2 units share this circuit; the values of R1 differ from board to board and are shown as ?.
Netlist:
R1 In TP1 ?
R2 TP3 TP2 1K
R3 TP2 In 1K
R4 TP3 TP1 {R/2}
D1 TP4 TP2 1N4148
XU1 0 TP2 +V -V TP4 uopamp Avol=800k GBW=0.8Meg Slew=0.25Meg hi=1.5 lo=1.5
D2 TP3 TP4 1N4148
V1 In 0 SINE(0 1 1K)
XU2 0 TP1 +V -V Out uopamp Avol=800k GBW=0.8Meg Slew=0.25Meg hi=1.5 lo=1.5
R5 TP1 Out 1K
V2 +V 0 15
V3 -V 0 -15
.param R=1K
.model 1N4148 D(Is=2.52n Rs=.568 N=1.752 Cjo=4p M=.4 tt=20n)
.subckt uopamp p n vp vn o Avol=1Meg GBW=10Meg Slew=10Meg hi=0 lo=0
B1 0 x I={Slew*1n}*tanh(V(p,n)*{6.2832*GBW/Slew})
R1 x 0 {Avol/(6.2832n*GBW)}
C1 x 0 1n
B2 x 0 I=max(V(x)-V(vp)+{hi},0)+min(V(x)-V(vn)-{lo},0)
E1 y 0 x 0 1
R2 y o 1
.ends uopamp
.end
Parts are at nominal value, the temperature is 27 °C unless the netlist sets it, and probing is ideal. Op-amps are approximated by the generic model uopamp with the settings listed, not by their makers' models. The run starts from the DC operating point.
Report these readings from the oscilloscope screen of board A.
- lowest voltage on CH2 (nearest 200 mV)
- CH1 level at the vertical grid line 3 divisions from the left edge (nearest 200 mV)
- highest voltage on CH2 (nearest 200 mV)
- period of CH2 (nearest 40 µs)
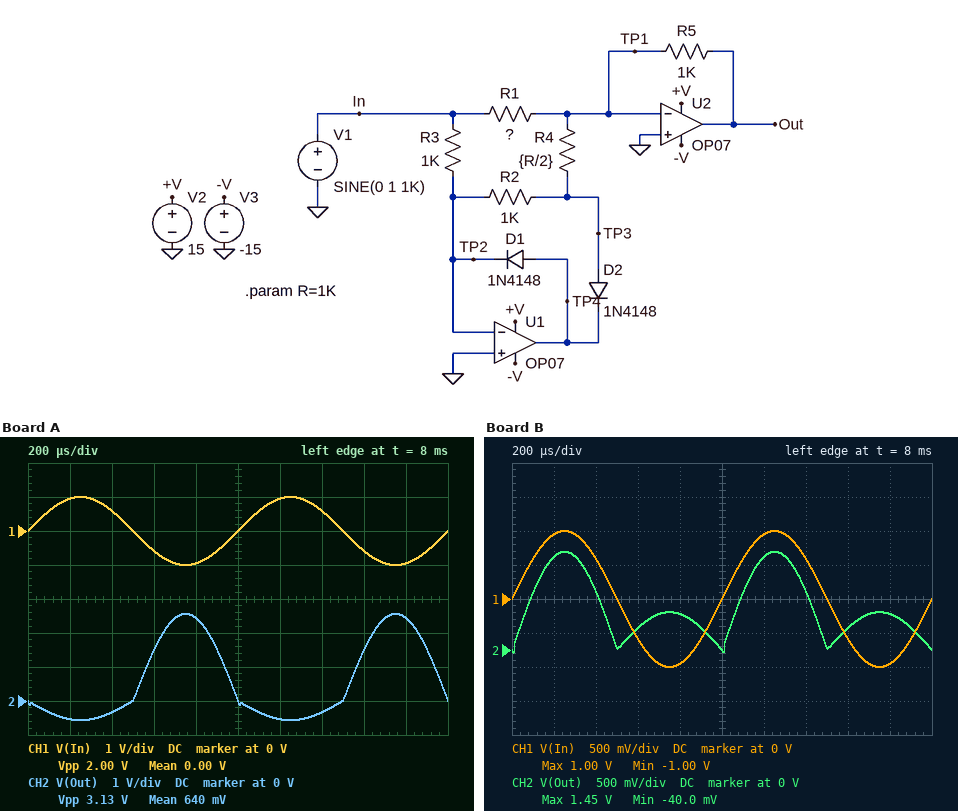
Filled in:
-600 mV
-600 mV
2.6 V
1.00 ms
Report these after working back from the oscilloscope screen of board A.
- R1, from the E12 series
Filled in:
390 Ω
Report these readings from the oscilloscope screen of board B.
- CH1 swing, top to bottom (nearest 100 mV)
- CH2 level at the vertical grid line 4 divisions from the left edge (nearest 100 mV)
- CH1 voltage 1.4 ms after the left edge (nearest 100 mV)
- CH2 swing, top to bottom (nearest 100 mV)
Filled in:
2.0 V
500 mV
600 mV
1.5 V
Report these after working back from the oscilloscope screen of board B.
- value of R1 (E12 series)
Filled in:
1.8 kΩ
